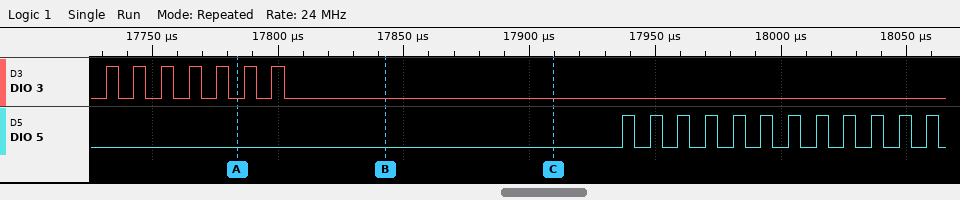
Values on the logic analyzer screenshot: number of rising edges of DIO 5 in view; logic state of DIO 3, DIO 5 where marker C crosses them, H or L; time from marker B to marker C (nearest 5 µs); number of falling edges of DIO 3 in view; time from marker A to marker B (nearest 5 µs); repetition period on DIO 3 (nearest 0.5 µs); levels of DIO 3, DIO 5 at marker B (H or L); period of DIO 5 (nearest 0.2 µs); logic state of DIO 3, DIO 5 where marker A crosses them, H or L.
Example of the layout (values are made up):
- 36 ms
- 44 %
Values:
- 12
- DIO 3=L, DIO 5=L
- 65 µs
- 7
- 60 µs
- 11 µs
- DIO 3=L, DIO 5=L
- 11 µs
- DIO 3=L, DIO 5=L
